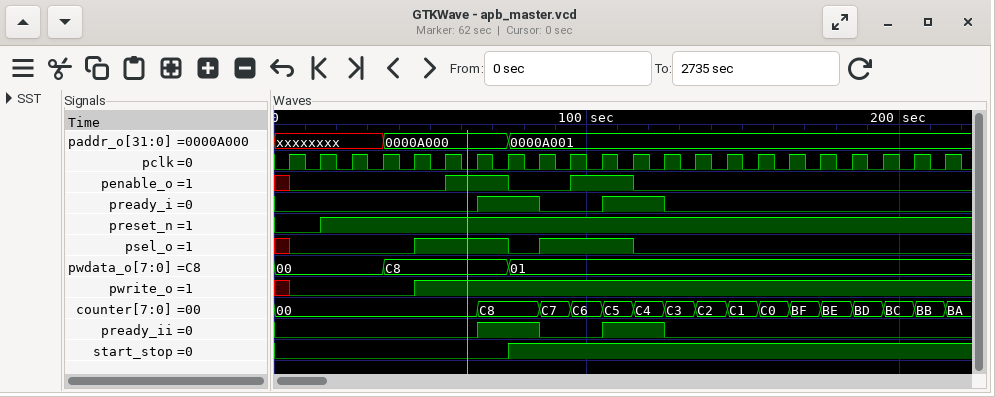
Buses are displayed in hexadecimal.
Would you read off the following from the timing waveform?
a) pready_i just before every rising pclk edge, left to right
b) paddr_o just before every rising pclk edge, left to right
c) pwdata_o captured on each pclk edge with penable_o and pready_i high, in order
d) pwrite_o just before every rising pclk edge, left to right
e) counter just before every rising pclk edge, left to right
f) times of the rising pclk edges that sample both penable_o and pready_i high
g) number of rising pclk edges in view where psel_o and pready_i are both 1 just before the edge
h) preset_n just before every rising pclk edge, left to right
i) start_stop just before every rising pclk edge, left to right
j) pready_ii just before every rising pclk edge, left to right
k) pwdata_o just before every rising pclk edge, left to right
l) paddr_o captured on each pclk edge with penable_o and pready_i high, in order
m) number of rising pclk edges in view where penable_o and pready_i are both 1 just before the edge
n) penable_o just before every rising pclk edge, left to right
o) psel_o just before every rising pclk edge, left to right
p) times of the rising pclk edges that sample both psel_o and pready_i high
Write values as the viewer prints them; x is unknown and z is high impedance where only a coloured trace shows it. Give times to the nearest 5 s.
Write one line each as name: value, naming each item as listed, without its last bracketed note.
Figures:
pready_i just before every rising pclk edge, left to right: 0 0 0 0 0 0 0 1 1 0 0 1 1 0 0 0 0 0 0 0 0 0
paddr_o just before every rising pclk edge, left to right: xxxxxxxx, xxxxxxxx, xxxxxxxx, xxxxxxxx, 0000A000, 0000A000, 0000A000, 0000A000, 0000A001, 0000A001, 0000A001, 0000A001, 0000A001, 0000A001, 0000A001, 0000A001, 0000A001, 0000A001, 0000A001, 0000A001, 0000A001, 0000A001
pwdata_o captured on each pclk edge with penable_o and pready_i high, in order: C8, 01
pwrite_o just before every rising pclk edge, left to right: x 0 0 0 0 1 1 1 1 1 1 1 1 1 1 1 1 1 1 1 1 1
counter just before every rising pclk edge, left to right: 00, 00, 00, 00, 00, 00, 00, C8, C8, C7, C6, C5, C4, C3, C2, C1, C0, BF, BE, BD, BC, BB
times of the rising pclk edges that sample both penable_o and pready_i high: 75 s, 115 s
number of rising pclk edges in view where psel_o and pready_i are both 1 just before the edge: 2
preset_n just before every rising pclk edge, left to right: 0 0 1 1 1 1 1 1 1 1 1 1 1 1 1 1 1 1 1 1 1 1
start_stop just before every rising pclk edge, left to right: 0 0 0 0 0 0 0 0 1 1 1 1 1 1 1 1 1 1 1 1 1 1
pready_ii just before every rising pclk edge, left to right: 0 0 0 0 0 0 0 1 1 0 0 1 1 0 0 0 0 0 0 0 0 0
pwdata_o just before every rising pclk edge, left to right: 00, 00, 00, 00, C8, C8, C8, C8, 01, 01, 01, 01, 01, 01, 01, 01, 01, 01, 01, 01, 01, 01
paddr_o captured on each pclk edge with penable_o and pready_i high, in order: 0000A000, 0000A001
number of rising pclk edges in view where penable_o and pready_i are both 1 just before the edge: 2
penable_o just before every rising pclk edge, left to right: x 0 0 0 0 0 1 1 0 0 1 1 0 0 0 0 0 0 0 0 0 0
psel_o just before every rising pclk edge, left to right: x 0 0 0 0 1 1 1 0 1 1 1 0 0 0 0 0 0 0 0 0 0
times of the rising pclk edges that sample both psel_o and pready_i high: 75 s, 115 s
